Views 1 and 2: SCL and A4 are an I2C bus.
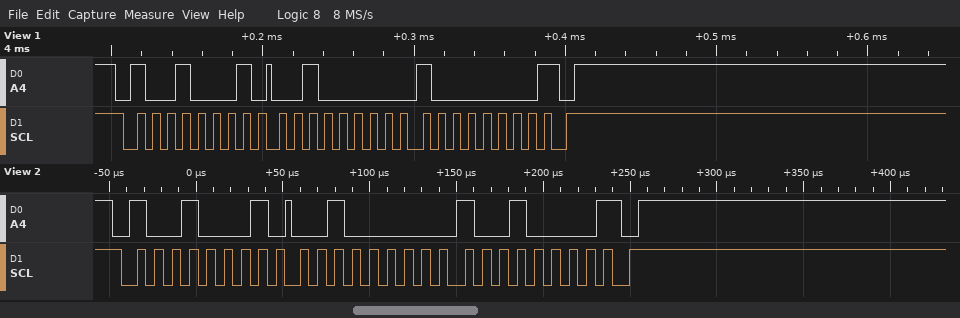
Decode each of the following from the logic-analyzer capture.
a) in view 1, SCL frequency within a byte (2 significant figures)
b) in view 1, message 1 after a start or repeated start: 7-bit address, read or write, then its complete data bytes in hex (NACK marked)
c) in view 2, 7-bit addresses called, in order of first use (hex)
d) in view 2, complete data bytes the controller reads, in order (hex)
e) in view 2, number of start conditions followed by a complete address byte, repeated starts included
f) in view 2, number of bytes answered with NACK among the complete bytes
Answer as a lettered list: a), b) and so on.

a) 100 kHz
b) 0x48 read: 20 80 NACK
c) 0x48
d) 20 90
e) 1
f) 1
